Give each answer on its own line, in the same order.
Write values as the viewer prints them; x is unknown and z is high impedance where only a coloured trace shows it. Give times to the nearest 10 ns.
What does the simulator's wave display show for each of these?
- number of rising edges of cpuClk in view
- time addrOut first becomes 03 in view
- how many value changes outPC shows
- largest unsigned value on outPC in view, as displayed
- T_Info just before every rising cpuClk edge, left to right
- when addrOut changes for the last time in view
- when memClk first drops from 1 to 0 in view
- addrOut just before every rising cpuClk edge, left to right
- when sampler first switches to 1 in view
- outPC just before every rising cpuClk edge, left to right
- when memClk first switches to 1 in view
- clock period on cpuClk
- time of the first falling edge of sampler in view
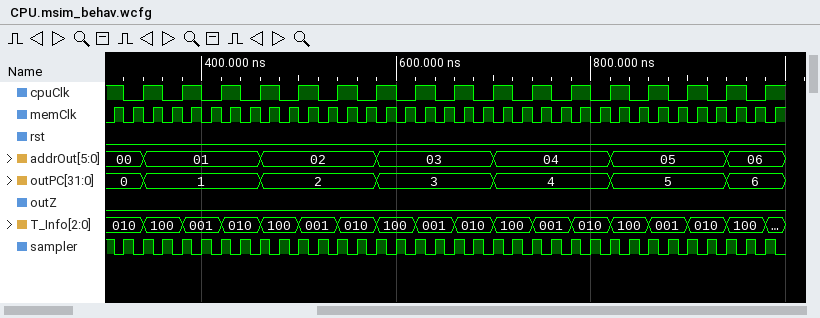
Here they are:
17
580 ns
6
6
010, 100, 001, 010, 100, 001, 010, 100, 001, 010, 100, 001, 010, 100, 001, 010, 100
940 ns
320 ns
00, 01, 01, 01, 02, 02, 02, 03, 03, 03, 04, 04, 04, 05, 05, 05, 06
320 ns
0, 1, 1, 1, 2, 2, 2, 3, 3, 3, 4, 4, 4, 5, 5, 5, 6
310 ns
40 ns
310 ns
